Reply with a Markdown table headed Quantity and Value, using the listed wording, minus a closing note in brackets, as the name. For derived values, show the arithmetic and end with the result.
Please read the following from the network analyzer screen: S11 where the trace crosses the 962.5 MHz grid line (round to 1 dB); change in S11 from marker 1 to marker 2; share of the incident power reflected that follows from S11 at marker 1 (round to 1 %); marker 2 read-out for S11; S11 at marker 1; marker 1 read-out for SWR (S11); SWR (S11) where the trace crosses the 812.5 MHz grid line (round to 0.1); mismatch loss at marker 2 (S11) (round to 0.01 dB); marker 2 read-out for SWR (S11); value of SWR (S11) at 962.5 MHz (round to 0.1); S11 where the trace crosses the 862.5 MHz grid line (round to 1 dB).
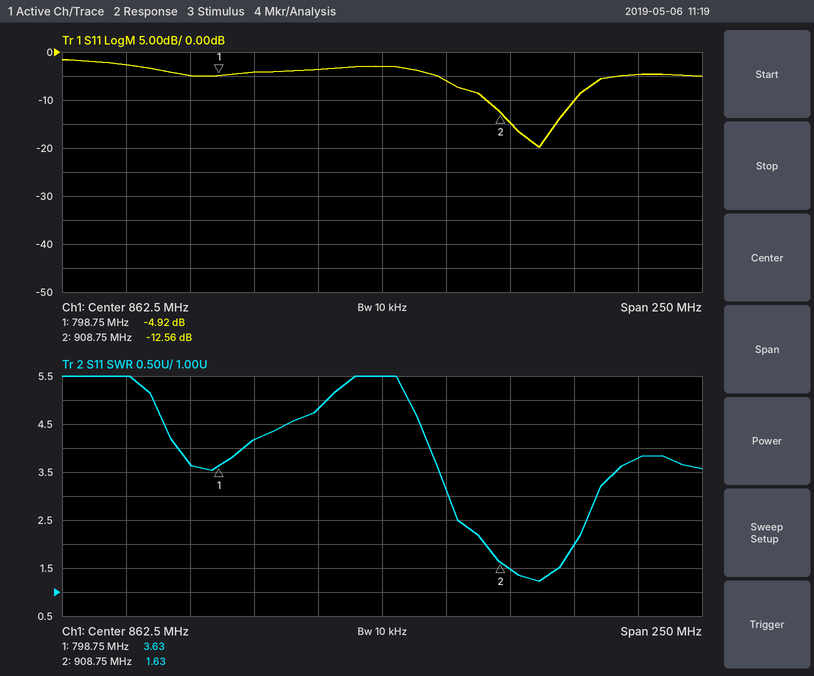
| Quantity | Value |
|---|---|
| S11 where the trace crosses the 962.5 MHz grid line | -5 dB |
| change in S11 from marker 1 to marker 2 | -12.56 − (-4.92) = -7.64 dB |
| share of the incident power reflected that follows from S11 at marker 1 | 10^(-4.92/10) ≈ 32 % |
| marker 2 read-out for S11 | -12.56 dB |
| S11 at marker 1 | -4.92 dB |
| marker 1 read-out for SWR | 3.63 |
| SWR (S11) where the trace crosses the 812.5 MHz grid line | 4.2 |
| mismatch loss at marker 2 (S11) | −10 log10(1 − 10^(-12.56/10)) ≈ 0.25 dB |
| marker 2 read-out for SWR | 1.63 |
| value of SWR (S11) at 962.5 MHz | 3.8 |
| S11 where the trace crosses the 862.5 MHz grid line | -3 dB |
